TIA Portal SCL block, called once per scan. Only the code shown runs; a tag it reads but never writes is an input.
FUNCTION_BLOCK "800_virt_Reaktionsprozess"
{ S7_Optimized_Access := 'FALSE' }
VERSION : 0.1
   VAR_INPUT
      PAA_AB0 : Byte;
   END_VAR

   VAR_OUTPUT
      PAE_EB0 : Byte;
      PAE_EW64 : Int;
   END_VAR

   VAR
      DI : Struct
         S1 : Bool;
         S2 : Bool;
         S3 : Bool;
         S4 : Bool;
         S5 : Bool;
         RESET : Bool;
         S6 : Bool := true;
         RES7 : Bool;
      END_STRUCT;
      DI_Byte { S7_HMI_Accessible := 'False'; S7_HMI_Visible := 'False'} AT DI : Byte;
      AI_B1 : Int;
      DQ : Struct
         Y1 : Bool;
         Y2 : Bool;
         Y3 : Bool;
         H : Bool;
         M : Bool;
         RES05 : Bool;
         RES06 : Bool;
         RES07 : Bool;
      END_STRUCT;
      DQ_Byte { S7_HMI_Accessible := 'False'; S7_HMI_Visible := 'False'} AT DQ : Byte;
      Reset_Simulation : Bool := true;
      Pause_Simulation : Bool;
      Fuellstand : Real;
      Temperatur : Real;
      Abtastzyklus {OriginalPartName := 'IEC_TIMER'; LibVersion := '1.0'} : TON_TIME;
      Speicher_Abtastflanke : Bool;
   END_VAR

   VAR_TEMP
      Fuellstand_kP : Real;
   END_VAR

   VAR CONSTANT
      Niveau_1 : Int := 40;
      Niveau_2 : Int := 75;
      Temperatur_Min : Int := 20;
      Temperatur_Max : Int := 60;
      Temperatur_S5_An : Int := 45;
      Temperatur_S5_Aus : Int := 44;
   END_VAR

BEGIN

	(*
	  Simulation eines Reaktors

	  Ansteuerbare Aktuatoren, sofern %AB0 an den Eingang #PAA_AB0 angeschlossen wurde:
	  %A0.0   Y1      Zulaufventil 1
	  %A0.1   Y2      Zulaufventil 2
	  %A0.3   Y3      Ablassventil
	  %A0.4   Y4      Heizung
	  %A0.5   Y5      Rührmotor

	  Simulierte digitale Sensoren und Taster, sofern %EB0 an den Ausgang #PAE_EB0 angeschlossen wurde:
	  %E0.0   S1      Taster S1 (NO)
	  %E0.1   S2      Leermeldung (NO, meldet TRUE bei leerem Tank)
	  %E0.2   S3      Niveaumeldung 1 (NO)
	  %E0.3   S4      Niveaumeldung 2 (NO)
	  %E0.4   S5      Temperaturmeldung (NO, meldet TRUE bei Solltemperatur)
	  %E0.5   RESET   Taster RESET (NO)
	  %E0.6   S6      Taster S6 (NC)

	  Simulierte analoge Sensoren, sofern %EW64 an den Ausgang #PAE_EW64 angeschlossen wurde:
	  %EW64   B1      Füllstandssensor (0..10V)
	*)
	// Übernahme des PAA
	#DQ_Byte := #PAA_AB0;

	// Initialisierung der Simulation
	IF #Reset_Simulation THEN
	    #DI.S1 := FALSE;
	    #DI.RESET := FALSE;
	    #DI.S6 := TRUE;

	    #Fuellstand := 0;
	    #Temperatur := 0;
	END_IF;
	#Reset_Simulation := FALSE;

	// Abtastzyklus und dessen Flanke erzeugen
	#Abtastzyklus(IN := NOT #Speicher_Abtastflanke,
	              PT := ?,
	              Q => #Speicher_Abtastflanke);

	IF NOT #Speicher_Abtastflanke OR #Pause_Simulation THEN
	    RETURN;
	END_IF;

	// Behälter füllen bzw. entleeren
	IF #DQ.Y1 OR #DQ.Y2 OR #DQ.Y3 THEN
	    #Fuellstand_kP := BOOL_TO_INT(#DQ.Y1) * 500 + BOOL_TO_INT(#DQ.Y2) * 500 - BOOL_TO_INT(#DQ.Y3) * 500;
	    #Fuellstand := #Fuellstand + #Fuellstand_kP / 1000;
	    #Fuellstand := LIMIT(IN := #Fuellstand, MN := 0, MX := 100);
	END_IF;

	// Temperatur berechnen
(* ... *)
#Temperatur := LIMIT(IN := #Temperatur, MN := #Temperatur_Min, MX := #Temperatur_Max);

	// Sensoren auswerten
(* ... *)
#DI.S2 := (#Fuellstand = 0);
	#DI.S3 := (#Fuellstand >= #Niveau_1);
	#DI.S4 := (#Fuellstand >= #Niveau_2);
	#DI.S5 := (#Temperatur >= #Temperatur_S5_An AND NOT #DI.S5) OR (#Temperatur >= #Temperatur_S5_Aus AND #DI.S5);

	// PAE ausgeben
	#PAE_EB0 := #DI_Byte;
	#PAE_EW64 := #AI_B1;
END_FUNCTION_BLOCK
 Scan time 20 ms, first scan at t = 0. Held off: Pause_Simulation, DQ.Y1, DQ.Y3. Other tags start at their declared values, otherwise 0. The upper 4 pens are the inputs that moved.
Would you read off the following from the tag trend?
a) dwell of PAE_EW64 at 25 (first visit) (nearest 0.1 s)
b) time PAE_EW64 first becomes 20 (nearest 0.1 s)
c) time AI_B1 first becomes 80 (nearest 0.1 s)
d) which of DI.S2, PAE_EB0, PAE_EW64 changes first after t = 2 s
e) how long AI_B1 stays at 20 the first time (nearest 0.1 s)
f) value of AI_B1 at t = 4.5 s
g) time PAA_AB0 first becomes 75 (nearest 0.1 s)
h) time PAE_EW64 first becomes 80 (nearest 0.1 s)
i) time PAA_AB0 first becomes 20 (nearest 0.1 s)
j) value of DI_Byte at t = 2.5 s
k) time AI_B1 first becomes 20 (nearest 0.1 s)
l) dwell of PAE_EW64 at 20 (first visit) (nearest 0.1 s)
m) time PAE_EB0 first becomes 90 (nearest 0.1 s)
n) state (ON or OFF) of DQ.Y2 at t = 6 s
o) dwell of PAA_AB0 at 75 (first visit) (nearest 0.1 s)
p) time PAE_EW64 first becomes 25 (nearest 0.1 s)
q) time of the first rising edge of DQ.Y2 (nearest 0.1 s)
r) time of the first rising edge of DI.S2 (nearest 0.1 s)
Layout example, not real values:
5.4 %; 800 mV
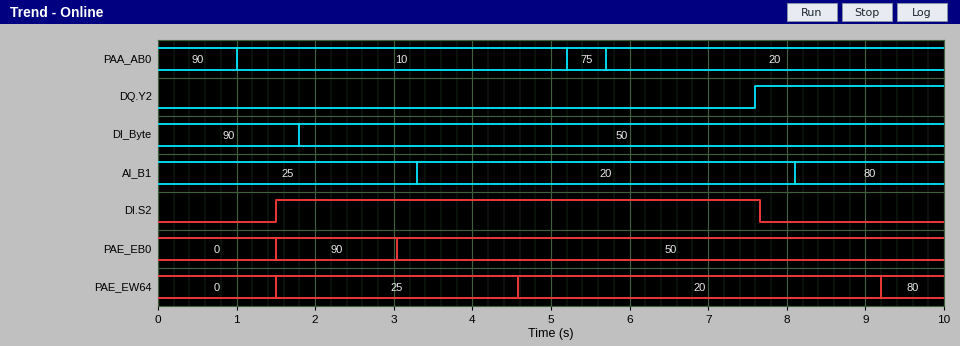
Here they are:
3.1 s; 4.6 s; 8.1 s; PAE_EB0; 4.8 s; 20; 5.2 s; 9.2 s; 5.7 s; 50; 3.3 s; 4.6 s; 1.5 s; OFF; 0.5 s; 1.5 s; 7.6 s; 1.5 s
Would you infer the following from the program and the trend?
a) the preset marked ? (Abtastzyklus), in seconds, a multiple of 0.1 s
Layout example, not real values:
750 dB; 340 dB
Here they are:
1.5 s
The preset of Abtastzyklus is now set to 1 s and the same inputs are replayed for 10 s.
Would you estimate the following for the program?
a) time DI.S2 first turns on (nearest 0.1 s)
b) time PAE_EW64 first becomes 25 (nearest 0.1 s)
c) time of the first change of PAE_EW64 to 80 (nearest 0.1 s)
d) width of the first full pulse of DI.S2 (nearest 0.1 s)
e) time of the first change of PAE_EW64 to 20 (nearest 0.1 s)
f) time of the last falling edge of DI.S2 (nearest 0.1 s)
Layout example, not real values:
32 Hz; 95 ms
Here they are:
1.0 s; 1.0 s; 8.3 s; 7.3 s; 4.1 s; 8.3 s
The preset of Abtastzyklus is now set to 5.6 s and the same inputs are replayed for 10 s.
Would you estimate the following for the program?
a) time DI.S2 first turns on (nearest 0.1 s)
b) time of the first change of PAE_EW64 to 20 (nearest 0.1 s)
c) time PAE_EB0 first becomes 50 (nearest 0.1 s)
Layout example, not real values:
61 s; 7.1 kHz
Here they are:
5.6 s; 5.6 s; 5.6 s
